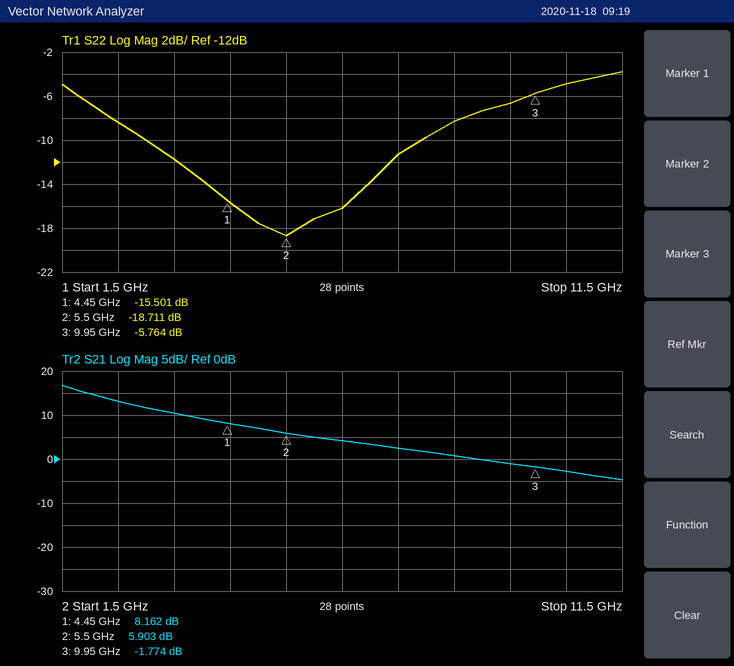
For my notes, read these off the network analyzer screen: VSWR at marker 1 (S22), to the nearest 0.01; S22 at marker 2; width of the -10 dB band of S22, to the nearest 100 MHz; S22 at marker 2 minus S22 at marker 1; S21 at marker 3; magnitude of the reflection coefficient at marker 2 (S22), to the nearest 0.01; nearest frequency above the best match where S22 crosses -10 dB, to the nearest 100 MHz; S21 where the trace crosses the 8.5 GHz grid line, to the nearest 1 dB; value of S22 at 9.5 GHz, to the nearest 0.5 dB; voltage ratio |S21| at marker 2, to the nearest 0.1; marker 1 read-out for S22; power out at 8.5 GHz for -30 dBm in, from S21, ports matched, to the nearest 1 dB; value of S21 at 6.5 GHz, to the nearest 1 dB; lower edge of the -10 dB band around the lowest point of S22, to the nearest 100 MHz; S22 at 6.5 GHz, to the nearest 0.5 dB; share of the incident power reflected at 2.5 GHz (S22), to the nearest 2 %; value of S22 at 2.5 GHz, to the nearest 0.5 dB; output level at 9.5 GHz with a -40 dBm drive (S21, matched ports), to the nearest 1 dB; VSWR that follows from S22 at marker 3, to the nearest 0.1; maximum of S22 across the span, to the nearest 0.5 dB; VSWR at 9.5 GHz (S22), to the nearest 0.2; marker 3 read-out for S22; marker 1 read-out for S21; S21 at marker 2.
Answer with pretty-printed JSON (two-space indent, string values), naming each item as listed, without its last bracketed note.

{
  "VSWR at marker 1 (S22), to the nearest 0.01": "1.40",
  "S22 at marker 2": "-18.711 dB",
  "width of the -10 dB band of S22, to the nearest 100 MHz": "4.9 GHz",
  "S22 at marker 2 minus S22 at marker 1": "-3.210 dB",
  "S21 at marker 3": "-1.774 dB",
  "magnitude of the reflection coefficient at marker 2 (S22), to the nearest 0.01": "0.12",
  "nearest frequency above the best match where S22 crosses -10 dB, to the nearest 100 MHz": "7.9 GHz",
  "S21 where the trace crosses the 8.5 GHz grid line, to the nearest 1 dB": "1 dB",
  "value of S22 at 9.5 GHz, to the nearest 0.5 dB": "-6.5 dB",
  "voltage ratio |S21| at marker 2, to the nearest 0.1": "2.0",
  "marker 1 read-out for S22": "-15.501 dB",
  "power out at 8.5 GHz for -30 dBm in, from S21, ports matched, to the nearest 1 dB": "-29 dBm",
  "value of S21 at 6.5 GHz, to the nearest 1 dB": "4 dB",
  "lower edge of the -10 dB band around the lowest point of S22, to the nearest 100 MHz": "3.0 GHz",
  "S22 at 6.5 GHz, to the nearest 0.5 dB": "-16.0 dB",
  "share of the incident power reflected at 2.5 GHz (S22), to the nearest 2 %": "14 %",
  "value of S22 at 2.5 GHz, to the nearest 0.5 dB": "-8.5 dB",
  "output level at 9.5 GHz with a -40 dBm drive (S21, matched ports), to the nearest 1 dB": "-41 dBm",
  "VSWR that follows from S22 at marker 3, to the nearest 0.1": "3.1",
  "maximum of S22 across the span, to the nearest 0.5 dB": "-4.0 dB",
  "VSWR at 9.5 GHz (S22), to the nearest 0.2": "2.8",
  "marker 3 read-out for S22": "-5.764 dB",
  "marker 1 read-out for S21": "8.162 dB",
  "S21 at marker 2": "5.903 dB"
}
